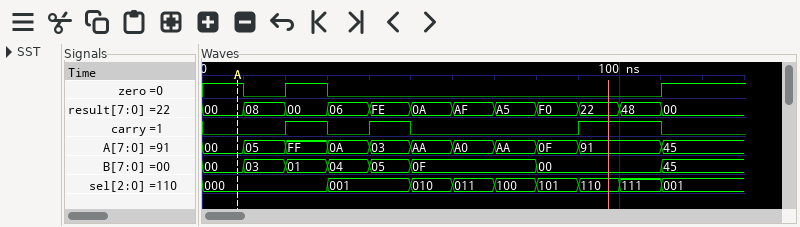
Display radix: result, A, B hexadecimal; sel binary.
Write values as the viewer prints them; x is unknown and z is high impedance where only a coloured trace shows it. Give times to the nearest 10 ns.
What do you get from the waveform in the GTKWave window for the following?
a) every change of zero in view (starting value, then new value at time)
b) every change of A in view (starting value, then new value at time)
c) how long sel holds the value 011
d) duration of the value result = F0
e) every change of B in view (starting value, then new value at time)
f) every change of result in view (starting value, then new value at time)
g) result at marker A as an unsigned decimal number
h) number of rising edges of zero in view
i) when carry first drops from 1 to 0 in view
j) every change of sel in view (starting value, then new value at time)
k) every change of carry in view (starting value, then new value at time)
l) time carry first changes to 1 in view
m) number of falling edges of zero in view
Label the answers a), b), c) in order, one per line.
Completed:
a) 1, 0 at 10 ns, 1 at 20 ns, 0 at 30 ns, 1 at 110 ns
b) 00, 05 at 10 ns, FF at 20 ns, 0A at 30 ns, 03 at 40 ns, AA at 50 ns, A0 at 60 ns, AA at 70 ns, 0F at 80 ns, 91 at 90 ns, 45 at 110 ns
c) 10 ns
d) 10 ns
e) 00, 03 at 10 ns, 01 at 20 ns, 04 at 30 ns, 05 at 40 ns, 0F at 50 ns, 00 at 80 ns, 45 at 110 ns
f) 00, 08 at 10 ns, 00 at 20 ns, 06 at 30 ns, FE at 40 ns, 0A at 50 ns, AF at 60 ns, A5 at 70 ns, F0 at 80 ns, 22 at 90 ns, 48 at 100 ns, 00 at 110 ns
g) 0
h) 2
i) 30 ns
j) 000, 001 at 30 ns, 010 at 50 ns, 011 at 60 ns, 100 at 70 ns, 101 at 80 ns, 110 at 90 ns, 111 at 100 ns, 001 at 110 ns
k) 0, 1 at 20 ns, 0 at 30 ns, 1 at 40 ns, 0 at 50 ns, 1 at 90 ns, 0 at 110 ns
l) 20 ns
m) 2
